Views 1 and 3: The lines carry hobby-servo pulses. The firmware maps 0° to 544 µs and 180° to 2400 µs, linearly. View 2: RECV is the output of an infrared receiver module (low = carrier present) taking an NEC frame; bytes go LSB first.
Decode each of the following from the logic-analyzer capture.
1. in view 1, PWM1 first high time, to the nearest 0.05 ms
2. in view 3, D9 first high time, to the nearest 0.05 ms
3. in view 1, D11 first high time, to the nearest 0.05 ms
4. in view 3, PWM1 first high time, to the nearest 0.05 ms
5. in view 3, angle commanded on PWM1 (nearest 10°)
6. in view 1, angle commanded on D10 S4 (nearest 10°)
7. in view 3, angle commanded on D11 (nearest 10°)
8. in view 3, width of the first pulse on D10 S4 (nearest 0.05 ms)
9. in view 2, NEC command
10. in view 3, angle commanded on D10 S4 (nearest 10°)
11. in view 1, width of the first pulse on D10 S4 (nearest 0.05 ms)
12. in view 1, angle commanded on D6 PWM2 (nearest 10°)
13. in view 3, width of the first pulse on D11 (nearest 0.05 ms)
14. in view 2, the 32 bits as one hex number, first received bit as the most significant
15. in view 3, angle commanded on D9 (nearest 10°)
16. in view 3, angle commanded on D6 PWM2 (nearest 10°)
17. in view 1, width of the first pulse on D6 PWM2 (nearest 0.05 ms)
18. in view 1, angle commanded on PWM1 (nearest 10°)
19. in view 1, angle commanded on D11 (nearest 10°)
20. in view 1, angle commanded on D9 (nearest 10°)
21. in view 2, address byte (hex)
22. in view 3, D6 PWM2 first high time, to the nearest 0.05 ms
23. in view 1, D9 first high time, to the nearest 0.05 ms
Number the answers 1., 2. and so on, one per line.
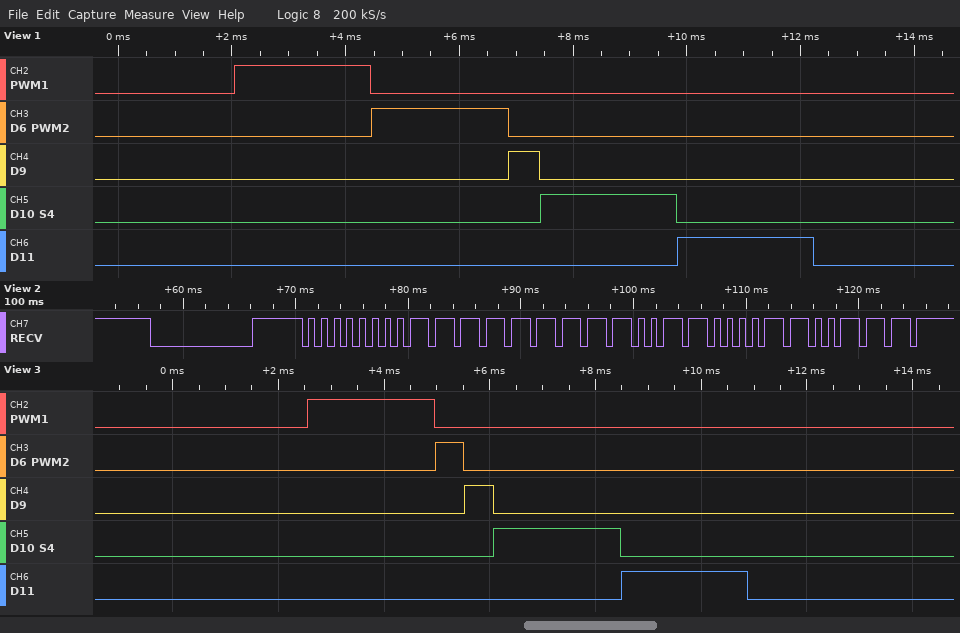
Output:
1. 2.40 ms
2. 0.55 ms
3. 2.40 ms
4. 2.40 ms
5. 180°
6. 180°
7. 180°
8. 2.40 ms
9. 0x19
10. 180°
11. 2.40 ms
12. 180°
13. 2.40 ms
14. 0x00FF9867
15. 0°
16. 0°
17. 2.40 ms
18. 180°
19. 180°
20. 0°
21. 0x00
22. 0.55 ms
23. 0.55 ms
